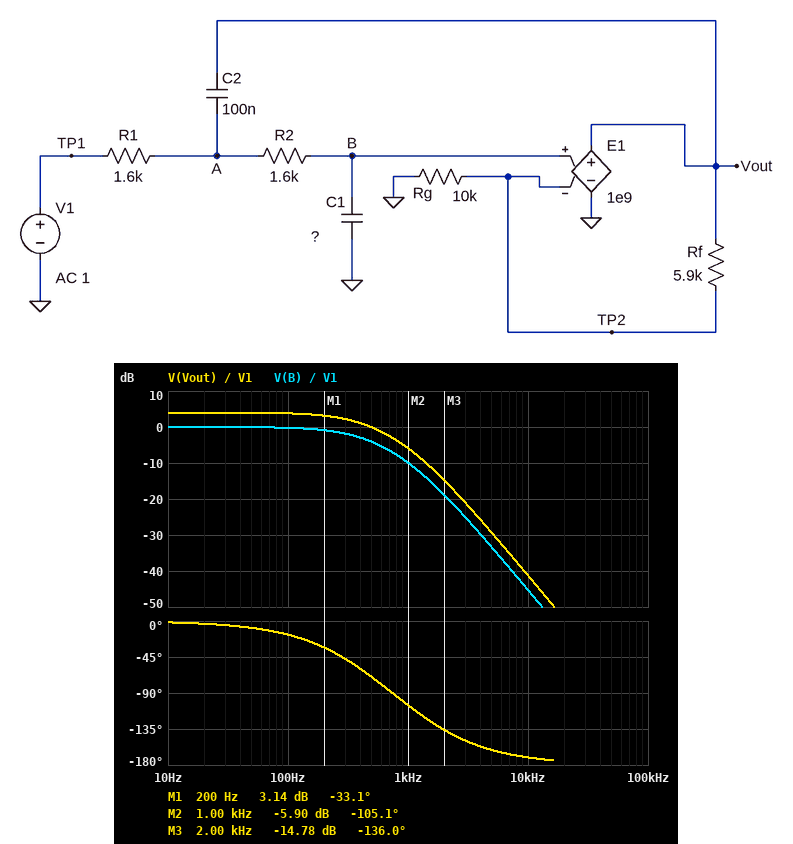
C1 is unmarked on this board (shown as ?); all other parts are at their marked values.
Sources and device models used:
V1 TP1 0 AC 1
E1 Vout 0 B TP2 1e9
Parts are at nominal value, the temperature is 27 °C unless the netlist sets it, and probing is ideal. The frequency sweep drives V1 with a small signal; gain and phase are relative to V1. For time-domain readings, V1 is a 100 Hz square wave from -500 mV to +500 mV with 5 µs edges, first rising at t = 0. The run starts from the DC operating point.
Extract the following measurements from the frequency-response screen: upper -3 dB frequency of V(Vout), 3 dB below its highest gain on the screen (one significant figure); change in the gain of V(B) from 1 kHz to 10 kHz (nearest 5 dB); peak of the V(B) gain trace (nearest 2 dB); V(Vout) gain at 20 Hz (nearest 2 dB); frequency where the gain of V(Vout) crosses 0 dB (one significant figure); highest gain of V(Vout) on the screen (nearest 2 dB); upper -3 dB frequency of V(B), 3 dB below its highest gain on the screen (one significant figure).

400 Hz
-35 dB
0 dB
4 dB
500 Hz
4 dB
400 Hz
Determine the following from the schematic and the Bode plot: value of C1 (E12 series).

180 nF
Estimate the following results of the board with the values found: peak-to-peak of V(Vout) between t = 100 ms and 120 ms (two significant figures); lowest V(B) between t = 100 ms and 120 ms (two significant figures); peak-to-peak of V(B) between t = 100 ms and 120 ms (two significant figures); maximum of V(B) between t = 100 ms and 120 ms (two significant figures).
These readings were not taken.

1.6 V
-500 mV
1.0 V
500 mV
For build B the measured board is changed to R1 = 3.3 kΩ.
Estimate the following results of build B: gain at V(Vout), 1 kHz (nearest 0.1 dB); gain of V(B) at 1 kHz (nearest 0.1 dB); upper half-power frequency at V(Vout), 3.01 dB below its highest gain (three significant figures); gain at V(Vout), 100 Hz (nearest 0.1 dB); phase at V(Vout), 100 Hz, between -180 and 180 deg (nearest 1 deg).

-10.2 dB
-14.2 dB
285 Hz
3.6 dB
-24 deg
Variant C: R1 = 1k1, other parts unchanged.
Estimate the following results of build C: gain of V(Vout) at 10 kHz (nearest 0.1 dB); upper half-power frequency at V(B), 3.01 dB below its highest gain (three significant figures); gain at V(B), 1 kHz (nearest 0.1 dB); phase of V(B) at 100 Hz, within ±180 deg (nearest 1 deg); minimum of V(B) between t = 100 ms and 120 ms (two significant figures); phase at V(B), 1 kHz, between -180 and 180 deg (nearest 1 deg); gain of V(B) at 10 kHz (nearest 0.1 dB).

-38.0 dB
455 Hz
-8.5 dB
-15 deg
-500 mV
-95 deg
-42.1 dB
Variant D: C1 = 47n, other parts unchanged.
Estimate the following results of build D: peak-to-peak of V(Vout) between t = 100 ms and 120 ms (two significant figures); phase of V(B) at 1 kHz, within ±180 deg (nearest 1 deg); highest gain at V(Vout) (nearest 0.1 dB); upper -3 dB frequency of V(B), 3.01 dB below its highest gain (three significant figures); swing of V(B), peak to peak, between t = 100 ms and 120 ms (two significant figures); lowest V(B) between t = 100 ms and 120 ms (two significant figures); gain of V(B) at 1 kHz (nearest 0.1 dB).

3.0 V
-34 deg
10.2 dB
1.69 kHz
1.9 V
-940 mV
4.0 dB
